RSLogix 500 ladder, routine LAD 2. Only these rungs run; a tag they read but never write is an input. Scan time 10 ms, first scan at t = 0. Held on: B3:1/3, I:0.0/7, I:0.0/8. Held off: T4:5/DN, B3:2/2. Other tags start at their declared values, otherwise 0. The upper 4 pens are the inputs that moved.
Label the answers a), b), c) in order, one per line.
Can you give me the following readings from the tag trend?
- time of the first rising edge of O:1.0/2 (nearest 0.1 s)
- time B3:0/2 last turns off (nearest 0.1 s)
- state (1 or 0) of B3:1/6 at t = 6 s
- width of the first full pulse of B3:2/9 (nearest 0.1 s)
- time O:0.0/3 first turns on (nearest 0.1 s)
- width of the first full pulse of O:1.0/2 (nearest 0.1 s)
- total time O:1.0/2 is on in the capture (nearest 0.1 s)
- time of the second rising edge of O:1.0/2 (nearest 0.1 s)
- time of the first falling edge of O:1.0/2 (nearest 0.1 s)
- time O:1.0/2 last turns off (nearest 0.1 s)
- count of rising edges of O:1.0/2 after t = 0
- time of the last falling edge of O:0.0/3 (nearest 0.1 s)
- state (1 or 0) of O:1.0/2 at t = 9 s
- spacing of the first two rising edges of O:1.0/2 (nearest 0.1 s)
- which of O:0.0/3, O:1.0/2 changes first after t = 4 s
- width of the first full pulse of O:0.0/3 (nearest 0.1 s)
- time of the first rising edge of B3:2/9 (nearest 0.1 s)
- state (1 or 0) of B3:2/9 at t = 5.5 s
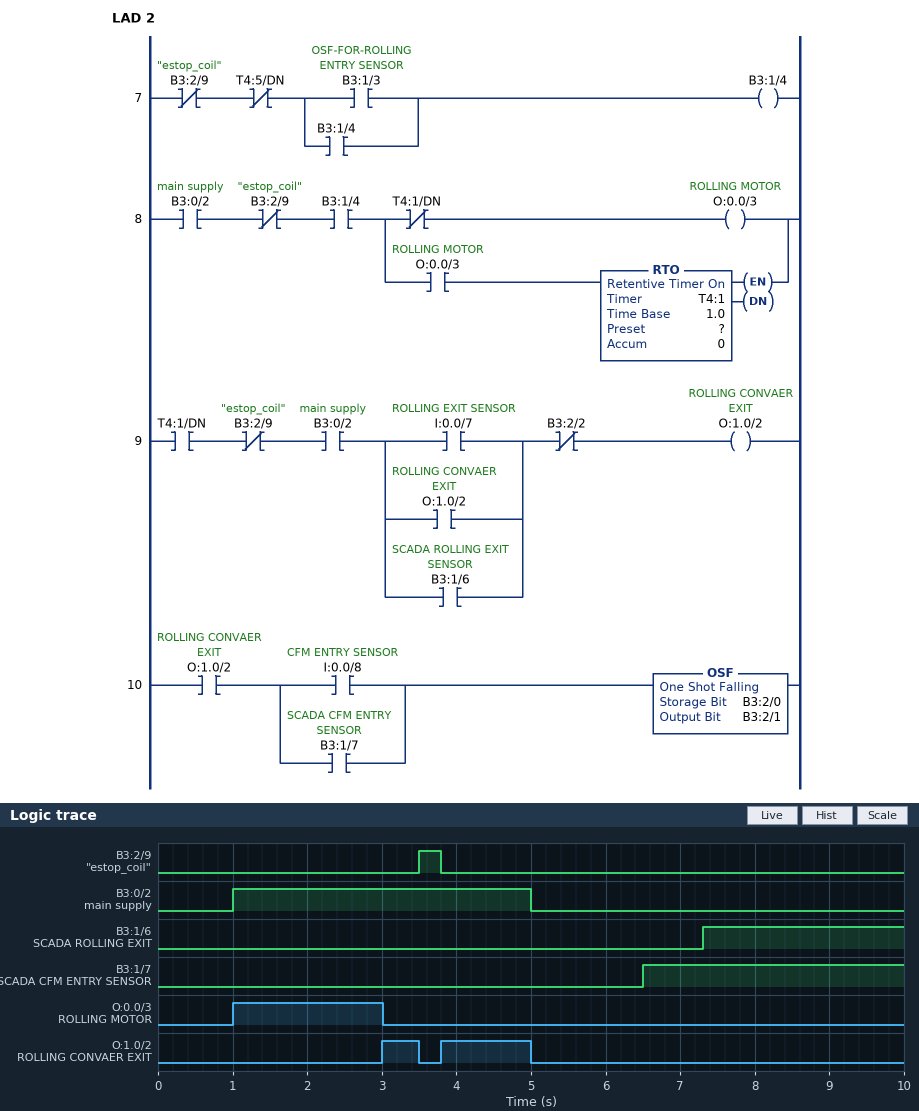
a) 3.0 s
b) 5.0 s
c) 0
d) 0.3 s
e) 1.0 s
f) 0.5 s
g) 1.7 s
h) 3.8 s
i) 3.5 s
j) 5.0 s
k) 2
l) 3.0 s
m) 0
n) 0.8 s
o) O:1.0/2
p) 2.0 s
q) 3.5 s
r) 0
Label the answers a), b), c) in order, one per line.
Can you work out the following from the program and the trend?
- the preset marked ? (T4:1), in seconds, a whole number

a) 2 s
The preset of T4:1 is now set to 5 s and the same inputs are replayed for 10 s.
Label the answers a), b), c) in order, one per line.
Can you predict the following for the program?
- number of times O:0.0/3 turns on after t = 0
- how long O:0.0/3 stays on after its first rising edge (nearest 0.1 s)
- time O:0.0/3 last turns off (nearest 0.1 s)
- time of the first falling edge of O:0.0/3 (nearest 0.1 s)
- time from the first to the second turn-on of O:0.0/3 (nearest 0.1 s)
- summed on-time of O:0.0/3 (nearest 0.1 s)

a) 2
b) 2.5 s
c) 5.0 s
d) 3.5 s
e) 2.8 s
f) 3.7 s
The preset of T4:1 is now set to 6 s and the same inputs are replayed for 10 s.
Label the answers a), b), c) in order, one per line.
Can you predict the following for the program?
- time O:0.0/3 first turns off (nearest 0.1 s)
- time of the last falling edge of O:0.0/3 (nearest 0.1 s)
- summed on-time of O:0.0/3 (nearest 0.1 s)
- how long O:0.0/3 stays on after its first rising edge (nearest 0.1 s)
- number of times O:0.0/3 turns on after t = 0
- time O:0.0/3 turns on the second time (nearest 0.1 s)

a) 3.5 s
b) 5.0 s
c) 3.7 s
d) 2.5 s
e) 2
f) 3.8 s
